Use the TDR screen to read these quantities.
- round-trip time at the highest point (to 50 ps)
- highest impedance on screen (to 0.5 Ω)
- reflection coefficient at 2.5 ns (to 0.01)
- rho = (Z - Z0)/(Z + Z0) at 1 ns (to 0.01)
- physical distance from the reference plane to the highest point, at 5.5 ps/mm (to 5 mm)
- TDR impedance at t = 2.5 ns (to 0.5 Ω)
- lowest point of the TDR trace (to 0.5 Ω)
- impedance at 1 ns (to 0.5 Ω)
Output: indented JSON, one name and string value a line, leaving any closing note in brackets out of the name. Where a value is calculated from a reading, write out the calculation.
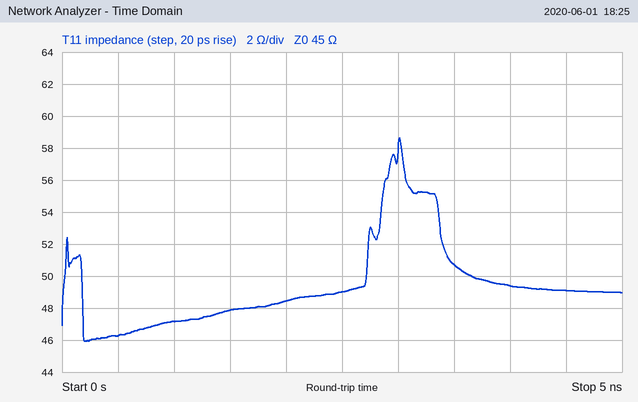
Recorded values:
{
  "round-trip time at the highest point": "3.00 ns",
  "highest impedance on screen": "58.5 Ω",
  "reflection coefficient at 2.5 ns": "(49 − 45)/(49 + 45) ≈ +0.04",
  "rho = (Z - Z0)/(Z + Z0) at 1 ns": "(47 − 45)/(47 + 45) ≈ +0.02",
  "physical distance from the reference plane to the highest point, at 5.5 ps/mm": "3.00 ns / 2 / 5.5 ps/mm ≈ 273 mm, so 275 mm to the nearest 5 mm",
  "TDR impedance at t = 2.5 ns": "49.0 Ω",
  "lowest point of the TDR trace": "46.0 Ω",
  "impedance at 1 ns": "47.0 Ω"
}
